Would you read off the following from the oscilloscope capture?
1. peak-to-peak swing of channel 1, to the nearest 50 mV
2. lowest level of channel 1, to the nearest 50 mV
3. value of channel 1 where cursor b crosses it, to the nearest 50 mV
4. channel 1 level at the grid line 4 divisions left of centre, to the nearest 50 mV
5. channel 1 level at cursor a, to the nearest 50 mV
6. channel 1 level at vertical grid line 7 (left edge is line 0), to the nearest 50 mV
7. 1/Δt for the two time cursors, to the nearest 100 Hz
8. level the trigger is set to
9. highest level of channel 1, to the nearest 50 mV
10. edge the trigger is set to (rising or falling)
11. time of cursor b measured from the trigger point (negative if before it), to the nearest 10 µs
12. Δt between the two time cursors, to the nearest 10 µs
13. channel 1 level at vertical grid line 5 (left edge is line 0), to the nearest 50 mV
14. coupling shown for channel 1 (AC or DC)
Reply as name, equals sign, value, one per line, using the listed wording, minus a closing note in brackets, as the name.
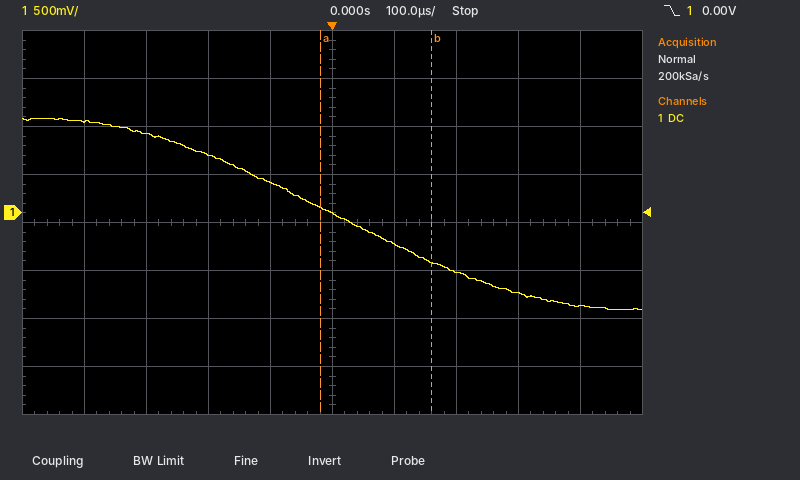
peak-to-peak swing of channel 1, to the nearest 50 mV = 2.00 V
lowest level of channel 1, to the nearest 50 mV = -1.00 V
value of channel 1 where cursor b crosses it, to the nearest 50 mV = -500 mV
channel 1 level at the grid line 4 divisions left of centre, to the nearest 50 mV = 950 mV
channel 1 level at cursor a, to the nearest 50 mV = 50 mV
channel 1 level at vertical grid line 7 (left edge is line 0), to the nearest 50 mV = -600 mV
1/Δt for the two time cursors, to the nearest 100 Hz = 5.6 kHz
level the trigger is set to = 0.00 V
highest level of channel 1, to the nearest 50 mV = 1.00 V
edge the trigger is set to = falling
time of cursor b measured from the trigger point (negative if before it), to the nearest 10 µs = +160 µs
Δt between the two time cursors, to the nearest 10 µs = 180 µs
channel 1 level at vertical grid line 5 (left edge is line 0), to the nearest 50 mV = 0 mV
coupling shown for channel 1 = DC
